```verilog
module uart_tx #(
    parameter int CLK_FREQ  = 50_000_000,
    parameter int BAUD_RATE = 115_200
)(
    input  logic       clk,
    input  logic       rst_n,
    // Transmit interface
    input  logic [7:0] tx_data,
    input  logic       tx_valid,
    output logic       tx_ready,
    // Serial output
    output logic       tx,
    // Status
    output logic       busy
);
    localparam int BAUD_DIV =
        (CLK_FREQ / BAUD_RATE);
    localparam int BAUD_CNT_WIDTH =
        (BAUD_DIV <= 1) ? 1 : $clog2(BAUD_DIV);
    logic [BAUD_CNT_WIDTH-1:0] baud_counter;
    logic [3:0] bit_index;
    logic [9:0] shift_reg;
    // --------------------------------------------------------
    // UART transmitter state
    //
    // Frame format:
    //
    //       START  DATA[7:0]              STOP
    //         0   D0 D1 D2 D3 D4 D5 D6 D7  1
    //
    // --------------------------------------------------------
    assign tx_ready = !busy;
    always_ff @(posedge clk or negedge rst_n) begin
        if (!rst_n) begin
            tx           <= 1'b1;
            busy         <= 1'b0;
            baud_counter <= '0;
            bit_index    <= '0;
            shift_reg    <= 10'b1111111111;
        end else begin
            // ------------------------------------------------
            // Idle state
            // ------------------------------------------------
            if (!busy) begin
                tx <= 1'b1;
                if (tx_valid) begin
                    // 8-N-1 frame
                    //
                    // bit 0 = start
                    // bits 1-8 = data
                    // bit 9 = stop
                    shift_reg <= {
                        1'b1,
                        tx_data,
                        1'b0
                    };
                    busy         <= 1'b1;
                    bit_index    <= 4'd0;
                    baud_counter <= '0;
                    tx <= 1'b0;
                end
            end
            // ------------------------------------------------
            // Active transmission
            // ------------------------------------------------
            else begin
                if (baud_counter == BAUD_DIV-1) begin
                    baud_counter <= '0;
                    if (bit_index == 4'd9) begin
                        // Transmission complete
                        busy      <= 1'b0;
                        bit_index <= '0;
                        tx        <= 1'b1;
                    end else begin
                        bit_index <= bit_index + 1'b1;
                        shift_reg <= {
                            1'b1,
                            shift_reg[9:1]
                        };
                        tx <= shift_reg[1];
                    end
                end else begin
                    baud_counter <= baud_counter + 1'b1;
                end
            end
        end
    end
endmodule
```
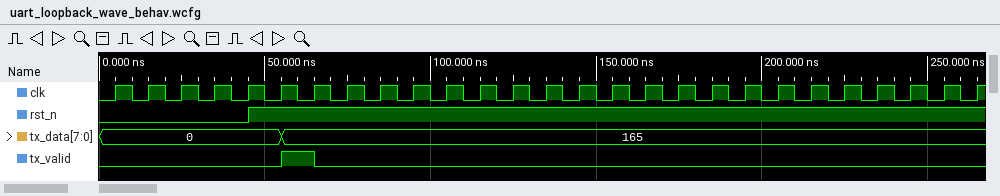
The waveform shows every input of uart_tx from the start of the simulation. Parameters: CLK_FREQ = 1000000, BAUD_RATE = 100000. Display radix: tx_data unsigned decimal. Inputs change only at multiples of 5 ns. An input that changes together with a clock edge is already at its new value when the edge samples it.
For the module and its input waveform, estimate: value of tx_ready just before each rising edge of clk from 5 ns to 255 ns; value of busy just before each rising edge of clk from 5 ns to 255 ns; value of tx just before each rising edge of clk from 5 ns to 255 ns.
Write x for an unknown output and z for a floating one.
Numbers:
1 1 1 1 1 1 0 0 0 0 0 0 0 0 0 0 0 0 0 0 0 0 0 0 0 0
0 0 0 0 0 0 1 1 1 1 1 1 1 1 1 1 1 1 1 1 1 1 1 1 1 1
1 1 1 1 1 1 0 0 0 0 0 0 0 0 0 0 1 1 1 1 1 1 1 1 1 1
